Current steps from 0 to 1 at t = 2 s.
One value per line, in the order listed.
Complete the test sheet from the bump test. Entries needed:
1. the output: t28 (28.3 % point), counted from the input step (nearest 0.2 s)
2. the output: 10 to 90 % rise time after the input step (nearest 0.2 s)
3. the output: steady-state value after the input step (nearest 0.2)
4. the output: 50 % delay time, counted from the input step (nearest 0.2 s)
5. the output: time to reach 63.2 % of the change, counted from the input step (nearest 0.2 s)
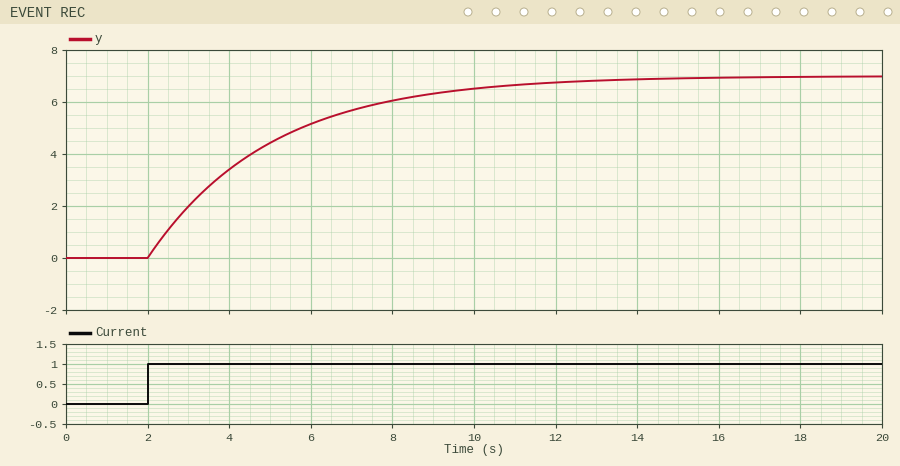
1.0 s
6.6 s
7.0
2.0 s
3.0 s
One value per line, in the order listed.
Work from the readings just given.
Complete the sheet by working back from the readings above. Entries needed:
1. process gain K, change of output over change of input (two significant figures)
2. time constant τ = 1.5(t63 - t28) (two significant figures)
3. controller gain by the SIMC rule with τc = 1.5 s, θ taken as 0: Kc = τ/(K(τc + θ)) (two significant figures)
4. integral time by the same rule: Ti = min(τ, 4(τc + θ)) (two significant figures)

7.0
3.0 s
0.29
3.0 s
